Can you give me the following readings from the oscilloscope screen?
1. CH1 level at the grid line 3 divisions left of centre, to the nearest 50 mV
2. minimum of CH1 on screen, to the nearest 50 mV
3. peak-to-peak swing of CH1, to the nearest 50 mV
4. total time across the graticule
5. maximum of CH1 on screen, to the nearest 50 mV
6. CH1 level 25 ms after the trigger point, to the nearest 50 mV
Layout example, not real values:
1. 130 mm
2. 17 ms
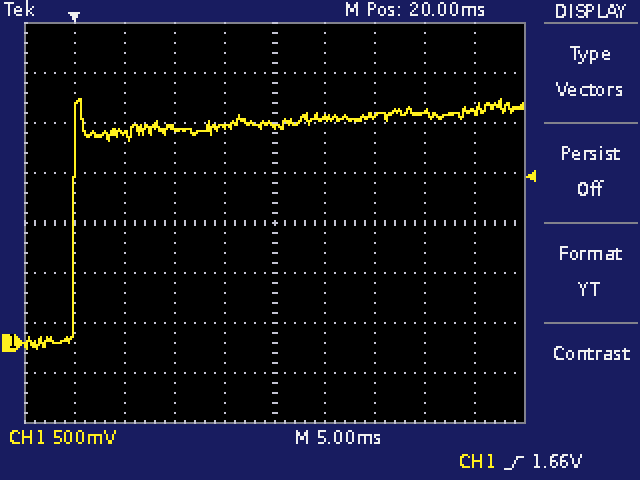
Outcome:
1. 2.10 V
2. -50 mV
3. 2.50 V
4. 50 ms
5. 2.45 V
6. 2.25 V
